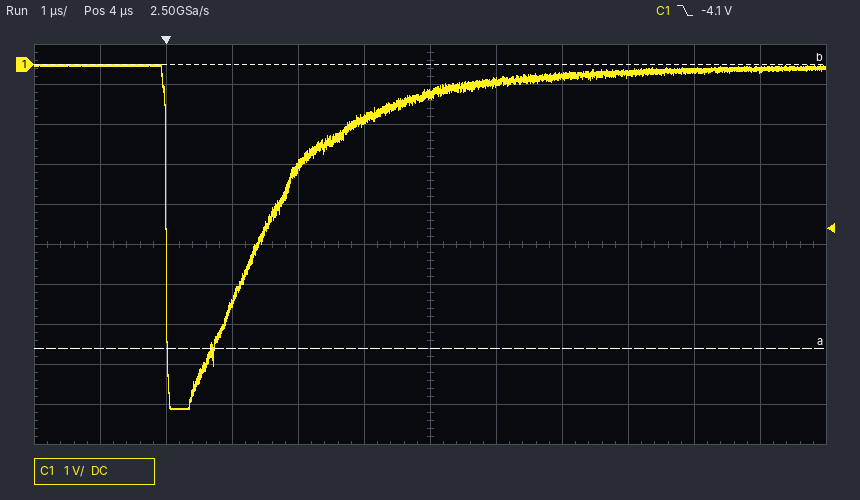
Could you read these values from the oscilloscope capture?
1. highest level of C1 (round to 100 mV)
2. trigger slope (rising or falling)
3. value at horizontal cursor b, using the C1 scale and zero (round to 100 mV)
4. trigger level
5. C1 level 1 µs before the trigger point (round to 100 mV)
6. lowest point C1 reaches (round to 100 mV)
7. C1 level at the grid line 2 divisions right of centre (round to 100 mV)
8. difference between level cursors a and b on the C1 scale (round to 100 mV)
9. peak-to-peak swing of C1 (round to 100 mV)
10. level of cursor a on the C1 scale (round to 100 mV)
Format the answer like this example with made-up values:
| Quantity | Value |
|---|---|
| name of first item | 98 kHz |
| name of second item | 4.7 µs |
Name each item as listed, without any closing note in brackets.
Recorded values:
| Quantity | Value |
|---|---|
| highest level of C1 | 0.0 V |
| trigger slope | falling |
| value at horizontal cursor b, using the C1 scale and zero | 0.0 V |
| trigger level | -4.1 V |
| C1 level 1 µs before the trigger point | 0.0 V |
| lowest point C1 reaches | -8.6 V |
| C1 level at the grid line 2 divisions right of centre | -300 mV |
| difference between level cursors a and b on the C1 scale | 7.1 V |
| peak-to-peak swing of C1 | 8.6 V |
| level of cursor a on the C1 scale | -7.1 V |
